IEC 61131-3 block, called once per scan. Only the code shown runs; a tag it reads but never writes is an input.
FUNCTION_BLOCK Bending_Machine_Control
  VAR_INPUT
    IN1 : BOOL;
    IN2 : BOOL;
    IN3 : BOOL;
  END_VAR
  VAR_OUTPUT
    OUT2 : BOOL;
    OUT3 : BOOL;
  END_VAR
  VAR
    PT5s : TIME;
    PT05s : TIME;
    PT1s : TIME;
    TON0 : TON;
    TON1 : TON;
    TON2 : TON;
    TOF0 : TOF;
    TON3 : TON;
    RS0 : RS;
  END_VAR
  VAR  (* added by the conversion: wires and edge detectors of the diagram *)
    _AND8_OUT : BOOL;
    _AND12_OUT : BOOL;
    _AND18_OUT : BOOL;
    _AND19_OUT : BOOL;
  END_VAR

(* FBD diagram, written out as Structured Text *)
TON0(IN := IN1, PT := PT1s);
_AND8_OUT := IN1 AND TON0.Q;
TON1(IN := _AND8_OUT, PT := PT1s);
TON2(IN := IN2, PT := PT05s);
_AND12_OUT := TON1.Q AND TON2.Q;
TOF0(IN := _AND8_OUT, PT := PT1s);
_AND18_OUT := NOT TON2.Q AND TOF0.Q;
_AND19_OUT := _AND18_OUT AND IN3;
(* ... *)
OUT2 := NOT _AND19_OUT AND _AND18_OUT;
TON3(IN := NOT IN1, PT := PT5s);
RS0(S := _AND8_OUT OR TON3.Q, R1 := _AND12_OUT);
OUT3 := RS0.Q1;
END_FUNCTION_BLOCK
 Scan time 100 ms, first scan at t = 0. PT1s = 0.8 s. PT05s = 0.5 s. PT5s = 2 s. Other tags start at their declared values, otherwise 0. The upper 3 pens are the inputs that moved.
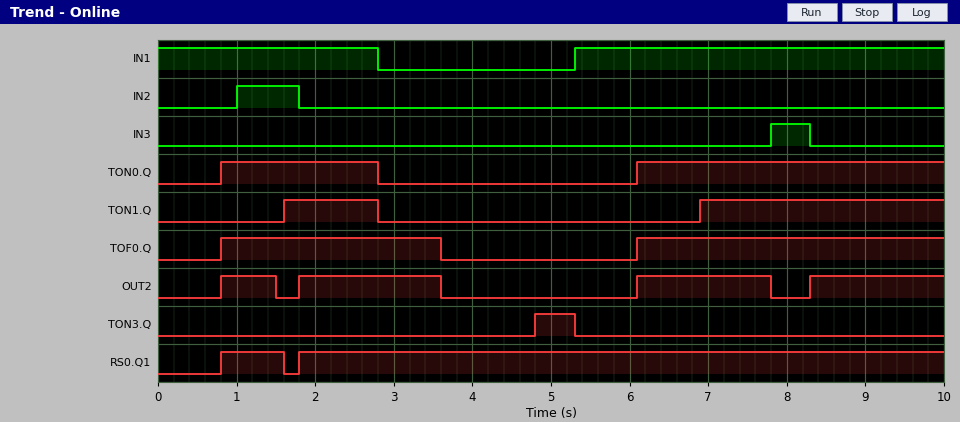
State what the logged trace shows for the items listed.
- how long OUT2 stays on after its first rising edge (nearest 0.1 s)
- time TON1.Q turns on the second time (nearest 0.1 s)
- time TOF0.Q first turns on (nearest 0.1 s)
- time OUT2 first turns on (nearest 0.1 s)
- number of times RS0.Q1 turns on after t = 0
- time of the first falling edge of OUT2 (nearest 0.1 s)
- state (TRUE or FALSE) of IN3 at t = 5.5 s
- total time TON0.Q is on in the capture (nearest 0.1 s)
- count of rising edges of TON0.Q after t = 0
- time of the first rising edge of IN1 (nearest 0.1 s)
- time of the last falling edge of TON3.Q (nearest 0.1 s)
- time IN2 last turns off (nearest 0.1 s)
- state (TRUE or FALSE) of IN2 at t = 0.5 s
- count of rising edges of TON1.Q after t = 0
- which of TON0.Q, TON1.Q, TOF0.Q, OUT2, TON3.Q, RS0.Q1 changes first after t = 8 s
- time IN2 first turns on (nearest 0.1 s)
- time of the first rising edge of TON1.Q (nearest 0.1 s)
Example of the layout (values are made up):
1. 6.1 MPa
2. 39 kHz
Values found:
1. 0.7 s
2. 6.9 s
3. 0.8 s
4. 0.8 s
5. 2
6. 1.5 s
7. FALSE
8. 5.9 s
9. 2
10. 5.3 s
11. 5.3 s
12. 1.8 s
13. FALSE
14. 2
15. OUT2
16. 1.0 s
17. 1.6 s
